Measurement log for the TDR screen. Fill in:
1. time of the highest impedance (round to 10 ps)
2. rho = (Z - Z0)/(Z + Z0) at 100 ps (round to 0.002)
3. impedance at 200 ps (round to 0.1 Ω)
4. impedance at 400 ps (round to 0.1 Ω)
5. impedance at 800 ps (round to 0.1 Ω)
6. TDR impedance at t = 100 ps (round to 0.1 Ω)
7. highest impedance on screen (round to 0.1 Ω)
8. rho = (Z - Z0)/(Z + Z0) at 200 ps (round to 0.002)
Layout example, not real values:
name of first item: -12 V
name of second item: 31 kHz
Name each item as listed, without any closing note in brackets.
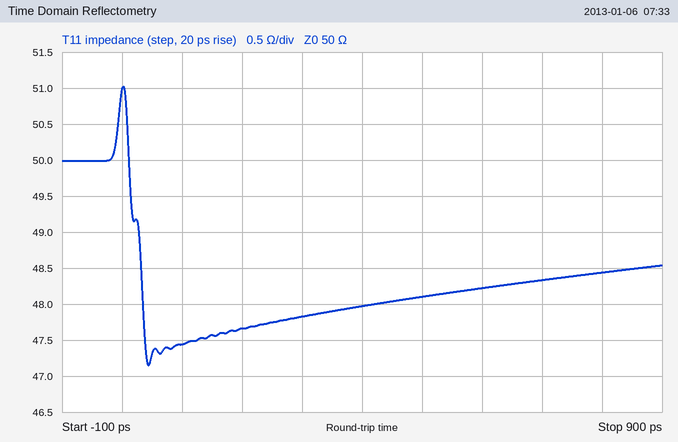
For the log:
time of the highest impedance: 0 ps
rho = (Z - Z0)/(Z + Z0) at 100 ps: -0.026
impedance at 200 ps: 47.7 Ω
impedance at 400 ps: 48.0 Ω
impedance at 800 ps: 48.4 Ω
TDR impedance at t = 100 ps: 47.4 Ω
highest impedance on screen: 51.0 Ω
rho = (Z - Z0)/(Z + Z0) at 200 ps: -0.024
